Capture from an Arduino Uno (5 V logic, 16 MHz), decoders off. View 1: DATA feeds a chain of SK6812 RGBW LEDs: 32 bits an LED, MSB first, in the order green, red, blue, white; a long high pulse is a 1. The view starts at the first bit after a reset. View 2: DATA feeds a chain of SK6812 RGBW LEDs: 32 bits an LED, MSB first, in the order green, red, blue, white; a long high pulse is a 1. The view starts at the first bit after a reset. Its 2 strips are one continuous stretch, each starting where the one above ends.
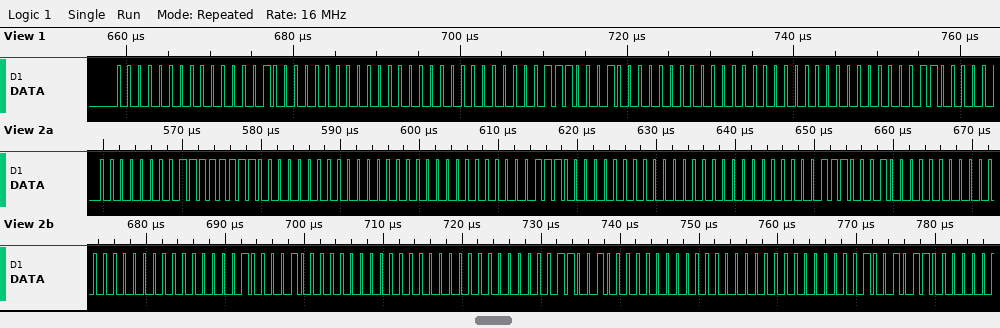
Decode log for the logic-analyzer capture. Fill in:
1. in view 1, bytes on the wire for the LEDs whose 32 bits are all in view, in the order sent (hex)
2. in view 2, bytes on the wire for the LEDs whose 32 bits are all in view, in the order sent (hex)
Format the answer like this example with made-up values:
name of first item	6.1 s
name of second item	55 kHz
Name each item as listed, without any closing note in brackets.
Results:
in view 1, bytes on the wire for the LEDs whose 32 bits are all in view, in the order sent	00 02 00 00 00 71 00 00
in view 2, bytes on the wire for the LEDs whose 32 bits are all in view, in the order sent	00 FF 00 00 00 0E 00 00 00 71 00 00 00 21 00 00 00 32 00 00
